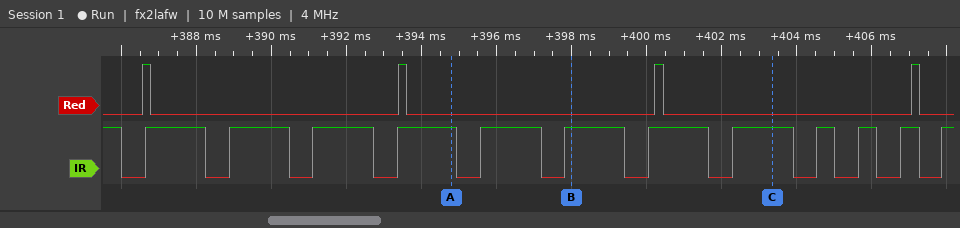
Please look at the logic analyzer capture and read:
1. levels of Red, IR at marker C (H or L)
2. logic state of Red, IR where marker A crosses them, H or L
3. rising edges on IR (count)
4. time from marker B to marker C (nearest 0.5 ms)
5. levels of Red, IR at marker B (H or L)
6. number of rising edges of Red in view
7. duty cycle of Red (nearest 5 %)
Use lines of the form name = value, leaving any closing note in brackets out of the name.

levels of Red, IR at marker C = Red=L, IR=H
logic state of Red, IR where marker A crosses them, H or L = Red=L, IR=H
rising edges on IR = 12
time from marker B to marker C = 5.5 ms
levels of Red, IR at marker B = Red=L, IR=H
number of rising edges of Red in view = 4
duty cycle of Red = 5 %
